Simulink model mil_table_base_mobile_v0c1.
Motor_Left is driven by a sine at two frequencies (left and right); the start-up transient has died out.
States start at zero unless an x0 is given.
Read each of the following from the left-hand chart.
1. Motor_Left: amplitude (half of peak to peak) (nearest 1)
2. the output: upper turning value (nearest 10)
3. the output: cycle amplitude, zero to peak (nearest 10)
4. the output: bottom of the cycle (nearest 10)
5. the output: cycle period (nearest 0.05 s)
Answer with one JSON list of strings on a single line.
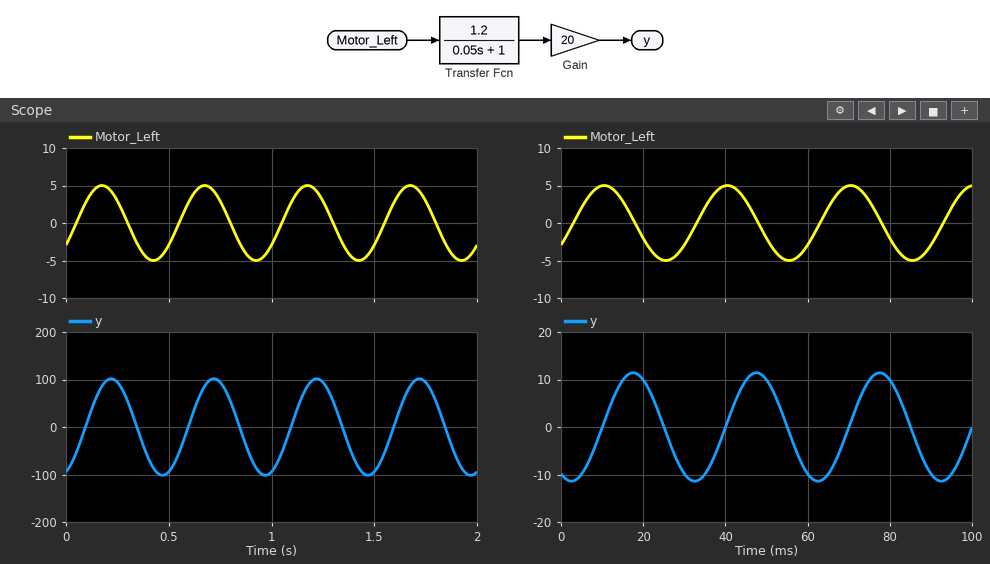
["5", "100", "100", "-100", "0.50 s"]
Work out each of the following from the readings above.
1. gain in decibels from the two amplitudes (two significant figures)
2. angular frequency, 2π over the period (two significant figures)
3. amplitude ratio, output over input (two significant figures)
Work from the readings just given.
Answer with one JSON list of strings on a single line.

["26 dB", "13 rad/s", "20"]
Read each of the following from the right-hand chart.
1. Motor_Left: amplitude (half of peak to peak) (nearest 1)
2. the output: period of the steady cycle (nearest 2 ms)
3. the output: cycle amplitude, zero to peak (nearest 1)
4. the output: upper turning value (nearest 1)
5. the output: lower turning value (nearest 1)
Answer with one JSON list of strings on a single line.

["5", "30 ms", "11", "11", "-11"]
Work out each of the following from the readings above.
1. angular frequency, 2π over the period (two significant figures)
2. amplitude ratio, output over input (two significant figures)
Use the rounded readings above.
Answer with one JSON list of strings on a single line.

["0.21 rad/ms", "2.2"]
